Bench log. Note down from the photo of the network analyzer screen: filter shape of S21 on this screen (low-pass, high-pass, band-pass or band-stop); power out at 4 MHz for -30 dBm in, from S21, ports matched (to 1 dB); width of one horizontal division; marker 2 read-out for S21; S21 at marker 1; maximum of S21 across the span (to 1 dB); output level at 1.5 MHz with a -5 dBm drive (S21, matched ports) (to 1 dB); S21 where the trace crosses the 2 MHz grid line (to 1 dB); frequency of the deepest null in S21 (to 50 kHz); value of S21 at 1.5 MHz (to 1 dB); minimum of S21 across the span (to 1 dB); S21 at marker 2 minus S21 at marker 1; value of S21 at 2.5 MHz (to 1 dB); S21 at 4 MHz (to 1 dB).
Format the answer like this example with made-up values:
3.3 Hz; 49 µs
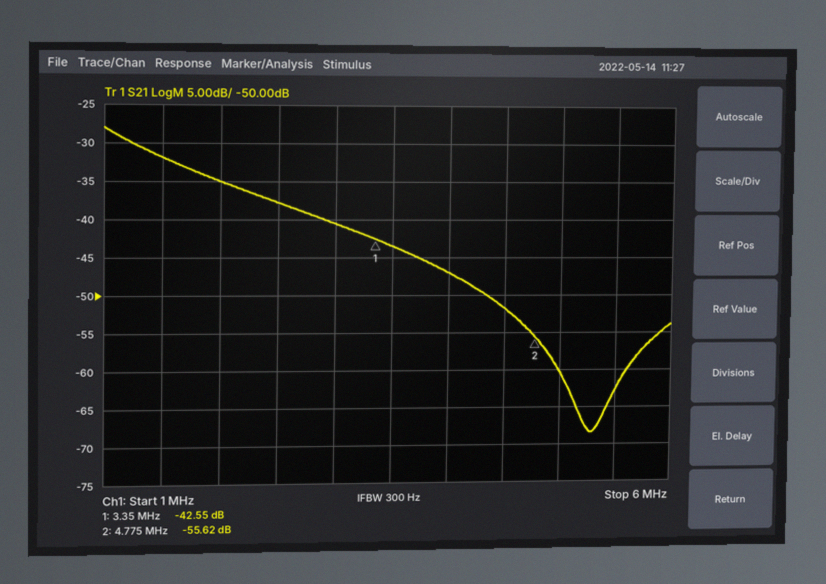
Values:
low-pass; -77 dBm; 500 kHz; -55.62 dB; -42.55 dB; -28 dB; -37 dBm; -35 dB; 5.30 MHz; -32 dB; -68 dB; -13.07 dB; -38 dB; -47 dB
